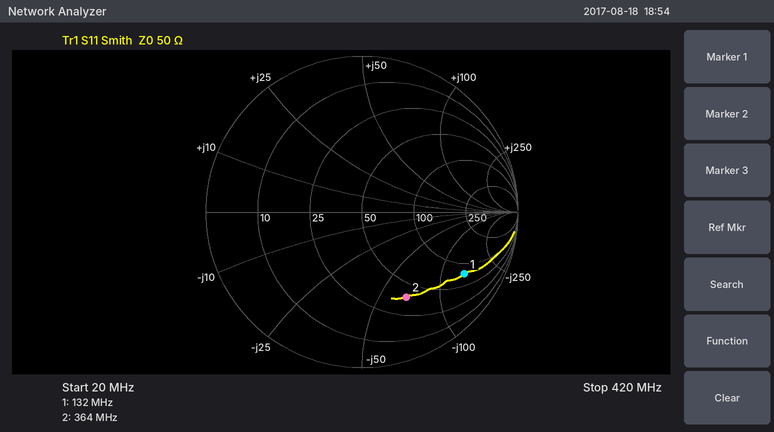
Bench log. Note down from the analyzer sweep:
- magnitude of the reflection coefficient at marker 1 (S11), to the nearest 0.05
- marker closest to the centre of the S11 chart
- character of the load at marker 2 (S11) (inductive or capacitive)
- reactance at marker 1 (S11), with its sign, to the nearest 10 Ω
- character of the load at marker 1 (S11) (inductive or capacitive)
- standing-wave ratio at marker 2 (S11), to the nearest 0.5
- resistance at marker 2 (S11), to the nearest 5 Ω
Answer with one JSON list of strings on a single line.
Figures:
["0.75", "marker 2", "capacitive", "-140 Ω", "capacitive", "4.0", "40 Ω"]
